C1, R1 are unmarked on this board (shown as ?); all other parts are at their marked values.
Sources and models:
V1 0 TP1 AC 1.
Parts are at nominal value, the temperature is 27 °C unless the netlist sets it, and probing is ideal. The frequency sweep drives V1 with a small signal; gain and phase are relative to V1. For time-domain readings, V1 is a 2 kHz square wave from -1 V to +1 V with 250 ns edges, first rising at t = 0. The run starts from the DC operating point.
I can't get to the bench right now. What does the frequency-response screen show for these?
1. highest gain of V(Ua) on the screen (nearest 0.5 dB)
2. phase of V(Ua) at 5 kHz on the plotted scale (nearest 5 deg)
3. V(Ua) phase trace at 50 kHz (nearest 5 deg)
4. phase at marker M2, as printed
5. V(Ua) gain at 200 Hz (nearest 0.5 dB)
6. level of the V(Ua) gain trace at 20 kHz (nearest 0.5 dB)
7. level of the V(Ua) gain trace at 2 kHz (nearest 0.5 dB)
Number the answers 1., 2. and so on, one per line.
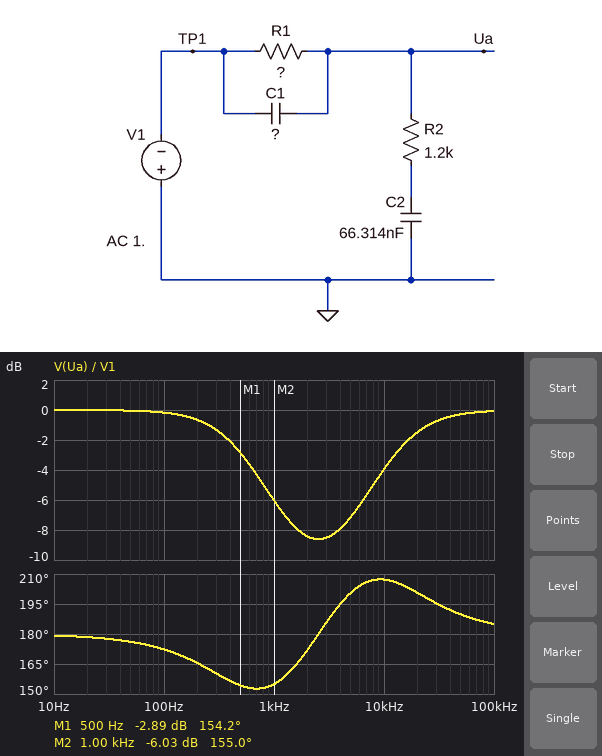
1. 0 dB
2. 200 deg
3. 190 deg
4. 155.0 deg
5. -0.5 dB
6. -1.5 dB
7. -8.5 dB
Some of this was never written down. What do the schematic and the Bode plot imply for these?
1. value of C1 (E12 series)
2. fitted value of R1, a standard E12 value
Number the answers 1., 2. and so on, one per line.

1. 15 nF
2. 3.3 kΩ
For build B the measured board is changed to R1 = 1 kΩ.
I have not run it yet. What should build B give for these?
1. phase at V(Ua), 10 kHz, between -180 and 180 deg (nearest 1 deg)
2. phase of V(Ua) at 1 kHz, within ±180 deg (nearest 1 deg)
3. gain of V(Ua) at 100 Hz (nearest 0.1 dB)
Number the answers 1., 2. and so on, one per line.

1. -168 deg
2. 165 deg
3. 0 dB
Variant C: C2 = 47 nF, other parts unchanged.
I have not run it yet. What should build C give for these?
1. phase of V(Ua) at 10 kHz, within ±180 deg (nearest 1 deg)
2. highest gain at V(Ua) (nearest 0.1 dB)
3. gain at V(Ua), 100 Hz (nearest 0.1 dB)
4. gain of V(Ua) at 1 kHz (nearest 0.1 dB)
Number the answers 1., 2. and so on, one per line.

1. -155 deg
2. 0 dB
3. -0.1 dB
4. -4.5 dB
